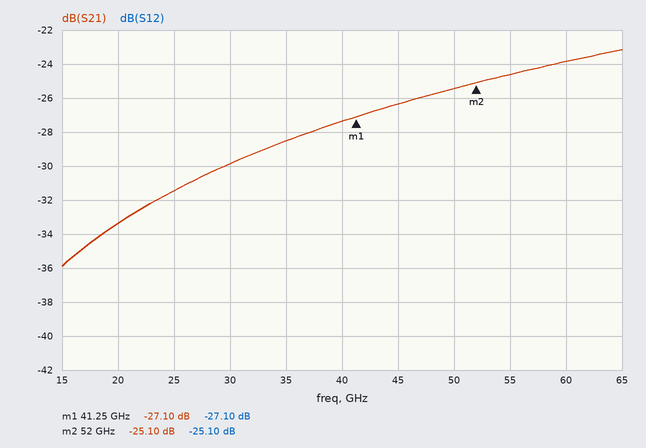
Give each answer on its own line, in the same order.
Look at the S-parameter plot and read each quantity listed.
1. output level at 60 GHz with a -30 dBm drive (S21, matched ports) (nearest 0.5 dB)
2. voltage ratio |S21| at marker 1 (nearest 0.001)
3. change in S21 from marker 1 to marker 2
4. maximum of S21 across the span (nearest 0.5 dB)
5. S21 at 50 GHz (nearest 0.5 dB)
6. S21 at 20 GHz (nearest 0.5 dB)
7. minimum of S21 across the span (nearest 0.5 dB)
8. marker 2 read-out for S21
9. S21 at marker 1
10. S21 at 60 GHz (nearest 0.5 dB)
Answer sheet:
-54.0 dBm
0.044
2.00 dB
-23.0 dB
-25.5 dB
-33.5 dB
-36.0 dB
-25.10 dB
-27.10 dB
-24.0 dB
